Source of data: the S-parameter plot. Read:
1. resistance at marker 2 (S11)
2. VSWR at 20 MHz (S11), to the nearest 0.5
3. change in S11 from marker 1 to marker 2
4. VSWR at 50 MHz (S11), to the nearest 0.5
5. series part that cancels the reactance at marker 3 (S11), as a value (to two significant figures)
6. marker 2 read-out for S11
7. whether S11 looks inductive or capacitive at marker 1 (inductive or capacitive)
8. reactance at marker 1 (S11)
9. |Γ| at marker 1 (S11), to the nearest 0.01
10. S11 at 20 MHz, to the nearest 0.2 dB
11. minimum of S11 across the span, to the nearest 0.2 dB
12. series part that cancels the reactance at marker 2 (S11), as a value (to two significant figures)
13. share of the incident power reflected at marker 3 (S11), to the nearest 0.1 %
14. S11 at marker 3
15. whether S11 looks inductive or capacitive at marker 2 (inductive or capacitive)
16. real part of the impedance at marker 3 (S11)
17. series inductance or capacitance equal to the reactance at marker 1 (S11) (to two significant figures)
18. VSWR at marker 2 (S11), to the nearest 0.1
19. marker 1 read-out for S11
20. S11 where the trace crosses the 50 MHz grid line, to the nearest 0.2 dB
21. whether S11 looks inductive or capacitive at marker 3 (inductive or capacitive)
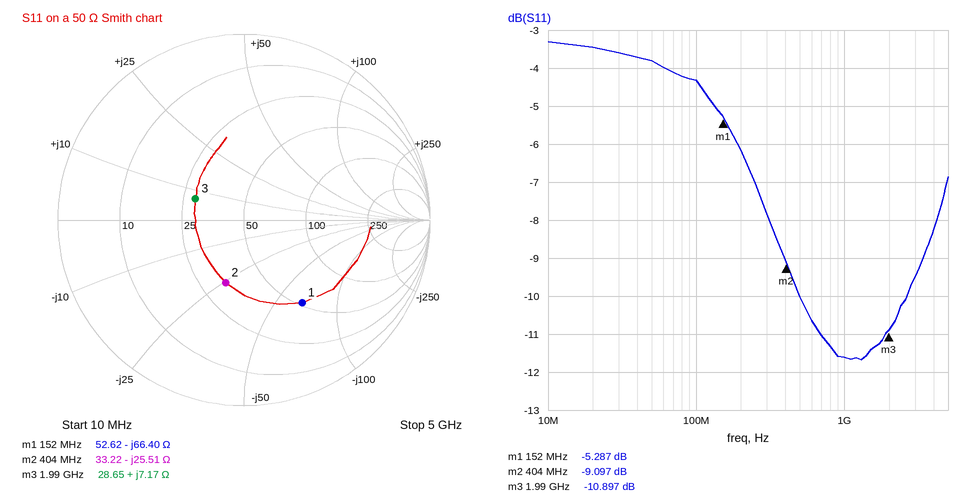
33.22 Ω
5.0
-3.810 dB
4.5
11 pF
-9.097 dB
capacitive
-66.40 Ω
0.54
-3.4 dB
-11.6 dB
10 nH
8.1 %
-10.897 dB
capacitive
28.65 Ω
16 pF
2.1
-5.287 dB
-3.8 dB
inductive
